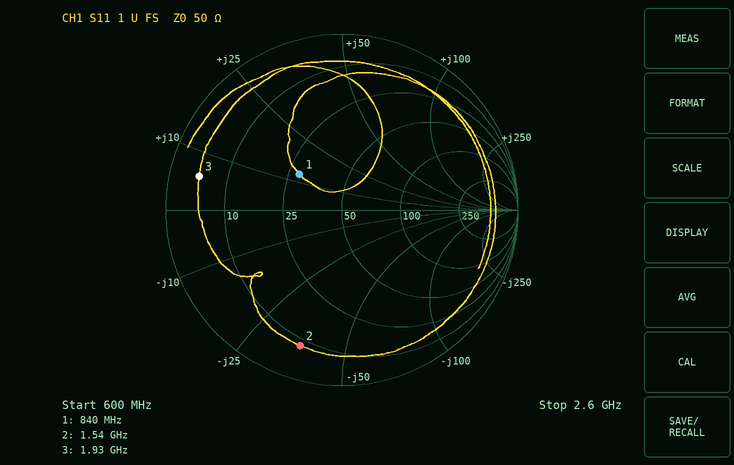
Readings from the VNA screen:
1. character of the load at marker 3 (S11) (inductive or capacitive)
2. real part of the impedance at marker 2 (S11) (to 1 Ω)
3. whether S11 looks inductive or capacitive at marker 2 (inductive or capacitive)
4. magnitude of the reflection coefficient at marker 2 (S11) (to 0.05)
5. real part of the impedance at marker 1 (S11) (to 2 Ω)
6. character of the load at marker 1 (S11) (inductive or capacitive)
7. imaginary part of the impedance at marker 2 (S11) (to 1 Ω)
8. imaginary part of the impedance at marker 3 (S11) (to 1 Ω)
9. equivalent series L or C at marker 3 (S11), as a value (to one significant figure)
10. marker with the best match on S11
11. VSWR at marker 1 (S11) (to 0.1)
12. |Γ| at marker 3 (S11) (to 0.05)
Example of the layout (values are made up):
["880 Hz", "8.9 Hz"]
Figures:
["inductive", "8 Ω", "capacitive", "0.80", "28 Ω", "inductive", "-36 Ω", "+6 Ω", "500 pH", "marker 1", "1.9", "0.85"]
